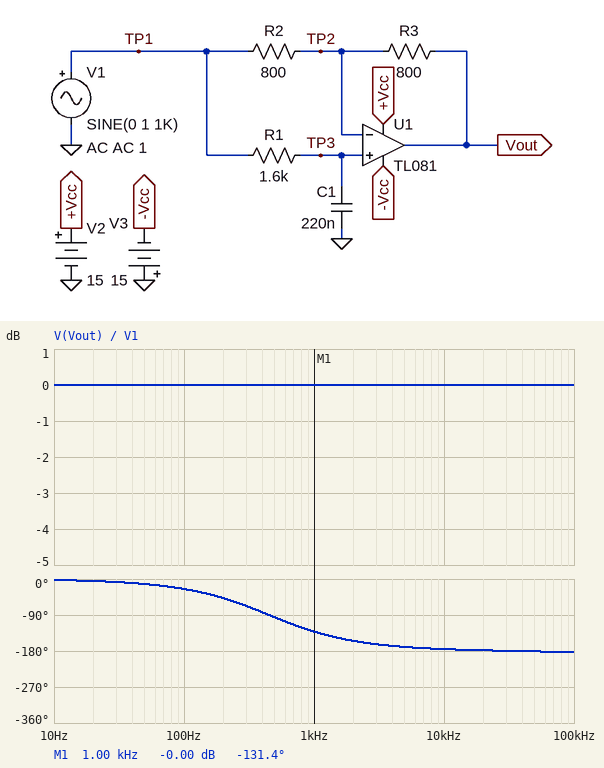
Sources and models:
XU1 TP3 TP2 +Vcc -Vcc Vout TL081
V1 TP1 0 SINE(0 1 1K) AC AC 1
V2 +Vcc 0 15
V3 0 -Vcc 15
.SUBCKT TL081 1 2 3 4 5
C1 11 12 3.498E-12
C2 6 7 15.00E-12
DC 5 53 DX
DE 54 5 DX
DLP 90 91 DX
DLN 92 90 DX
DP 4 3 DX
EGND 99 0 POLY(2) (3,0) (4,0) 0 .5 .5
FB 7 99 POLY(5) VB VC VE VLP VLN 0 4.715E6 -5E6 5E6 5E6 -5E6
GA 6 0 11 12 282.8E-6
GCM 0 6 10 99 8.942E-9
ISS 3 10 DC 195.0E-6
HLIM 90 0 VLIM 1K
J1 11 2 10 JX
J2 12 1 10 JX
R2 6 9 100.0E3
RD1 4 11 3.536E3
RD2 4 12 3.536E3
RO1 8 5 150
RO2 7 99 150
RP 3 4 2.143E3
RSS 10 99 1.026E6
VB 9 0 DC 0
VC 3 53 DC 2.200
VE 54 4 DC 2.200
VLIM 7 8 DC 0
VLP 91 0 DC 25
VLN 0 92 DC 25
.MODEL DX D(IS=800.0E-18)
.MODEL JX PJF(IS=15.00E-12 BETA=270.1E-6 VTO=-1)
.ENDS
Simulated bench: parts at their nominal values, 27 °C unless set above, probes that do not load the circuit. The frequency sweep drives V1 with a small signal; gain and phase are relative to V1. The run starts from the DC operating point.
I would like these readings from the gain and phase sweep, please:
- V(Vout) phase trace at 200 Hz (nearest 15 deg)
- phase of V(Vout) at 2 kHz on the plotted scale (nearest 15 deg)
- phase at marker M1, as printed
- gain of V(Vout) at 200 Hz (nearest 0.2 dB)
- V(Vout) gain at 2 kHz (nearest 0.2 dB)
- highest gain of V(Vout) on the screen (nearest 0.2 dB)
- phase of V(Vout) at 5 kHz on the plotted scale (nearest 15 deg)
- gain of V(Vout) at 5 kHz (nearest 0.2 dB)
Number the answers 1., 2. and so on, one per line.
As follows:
1. -45 deg
2. -150 deg
3. -131.4 deg
4. 0 dB
5. 0 dB
6. 0 dB
7. -165 deg
8. 0 dB
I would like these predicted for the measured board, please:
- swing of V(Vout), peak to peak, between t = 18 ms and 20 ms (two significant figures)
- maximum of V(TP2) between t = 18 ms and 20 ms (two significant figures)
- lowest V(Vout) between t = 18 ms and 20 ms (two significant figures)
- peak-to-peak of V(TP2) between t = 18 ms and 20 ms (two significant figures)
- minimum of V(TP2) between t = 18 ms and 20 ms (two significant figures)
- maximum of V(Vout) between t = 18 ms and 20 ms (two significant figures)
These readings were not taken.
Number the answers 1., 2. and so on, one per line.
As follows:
1. 2.0 V
2. 410 mV
3. -1.0 V
4. 820 mV
5. -410 mV
6. 1.0 V
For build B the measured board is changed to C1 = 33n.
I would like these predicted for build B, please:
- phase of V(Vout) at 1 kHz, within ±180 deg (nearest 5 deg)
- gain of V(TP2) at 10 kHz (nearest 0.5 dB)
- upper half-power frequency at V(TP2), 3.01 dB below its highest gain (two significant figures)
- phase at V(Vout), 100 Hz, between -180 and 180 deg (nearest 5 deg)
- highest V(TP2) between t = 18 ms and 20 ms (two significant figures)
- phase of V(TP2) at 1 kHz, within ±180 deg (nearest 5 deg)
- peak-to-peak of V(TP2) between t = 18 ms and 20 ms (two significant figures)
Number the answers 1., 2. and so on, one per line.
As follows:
1. -35 deg
2. -11.0 dB
3. 3.0 kHz
4. -5 deg
5. 950 mV
6. -20 deg
7. 1.9 V
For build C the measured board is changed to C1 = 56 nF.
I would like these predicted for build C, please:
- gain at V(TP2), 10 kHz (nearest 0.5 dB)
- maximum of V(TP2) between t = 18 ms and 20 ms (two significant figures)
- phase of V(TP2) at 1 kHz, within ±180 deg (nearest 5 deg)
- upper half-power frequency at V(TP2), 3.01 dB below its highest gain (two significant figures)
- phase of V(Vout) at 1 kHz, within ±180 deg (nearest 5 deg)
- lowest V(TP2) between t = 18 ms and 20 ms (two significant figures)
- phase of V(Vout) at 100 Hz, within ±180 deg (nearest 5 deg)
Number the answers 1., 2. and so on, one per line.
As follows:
1. -15.5 dB
2. 870 mV
3. -30 deg
4. 1.8 kHz
5. -60 deg
6. -870 mV
7. -5 deg
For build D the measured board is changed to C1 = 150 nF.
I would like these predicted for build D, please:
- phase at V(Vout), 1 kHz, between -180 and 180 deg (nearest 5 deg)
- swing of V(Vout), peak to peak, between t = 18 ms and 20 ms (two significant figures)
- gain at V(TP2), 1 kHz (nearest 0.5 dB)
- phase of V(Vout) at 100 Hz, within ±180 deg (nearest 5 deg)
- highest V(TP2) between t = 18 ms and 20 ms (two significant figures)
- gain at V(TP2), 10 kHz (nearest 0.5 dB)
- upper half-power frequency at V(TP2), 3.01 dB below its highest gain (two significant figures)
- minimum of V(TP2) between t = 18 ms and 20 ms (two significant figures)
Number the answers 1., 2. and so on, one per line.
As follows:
1. -115 deg
2. 2.0 V
3. -5.0 dB
4. -15 deg
5. 550 mV
6. -24.0 dB
7. 660 Hz
8. -550 mV
